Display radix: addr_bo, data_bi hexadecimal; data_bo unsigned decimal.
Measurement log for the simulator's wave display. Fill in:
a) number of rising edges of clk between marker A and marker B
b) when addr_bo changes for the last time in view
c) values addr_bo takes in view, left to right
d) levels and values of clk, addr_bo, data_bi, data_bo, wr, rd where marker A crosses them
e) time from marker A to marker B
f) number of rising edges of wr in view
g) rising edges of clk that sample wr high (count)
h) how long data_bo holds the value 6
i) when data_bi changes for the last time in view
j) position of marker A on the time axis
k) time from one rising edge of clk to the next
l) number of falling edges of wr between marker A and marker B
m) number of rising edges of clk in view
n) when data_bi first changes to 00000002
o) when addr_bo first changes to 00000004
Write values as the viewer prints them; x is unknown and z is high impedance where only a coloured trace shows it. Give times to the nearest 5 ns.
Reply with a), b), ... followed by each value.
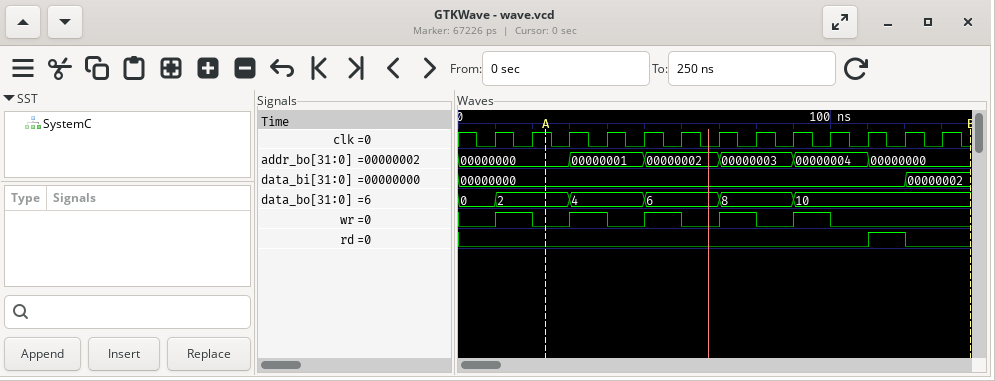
a) 11
b) 110 ns
c) 00000000, 00000001, 00000002, 00000003, 00000004, 00000000
d) clk=1, addr_bo=00000000, data_bi=00000000, data_bo=2, wr=0, rd=0
e) 115 ns
f) 5
g) 5
h) 20 ns
i) 120 ns
j) 25 ns
k) 10 ns
l) 4
m) 13
n) 120 ns
o) 90 ns
